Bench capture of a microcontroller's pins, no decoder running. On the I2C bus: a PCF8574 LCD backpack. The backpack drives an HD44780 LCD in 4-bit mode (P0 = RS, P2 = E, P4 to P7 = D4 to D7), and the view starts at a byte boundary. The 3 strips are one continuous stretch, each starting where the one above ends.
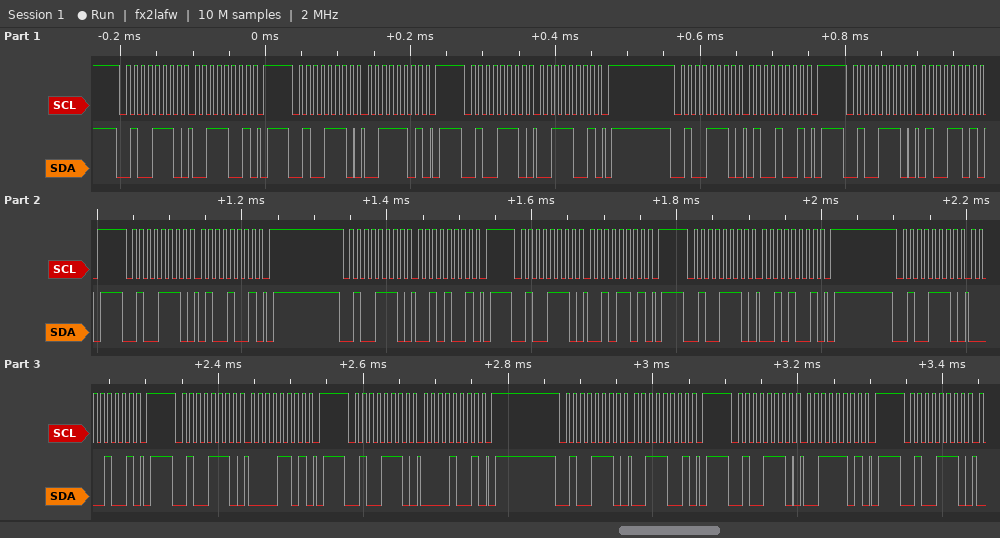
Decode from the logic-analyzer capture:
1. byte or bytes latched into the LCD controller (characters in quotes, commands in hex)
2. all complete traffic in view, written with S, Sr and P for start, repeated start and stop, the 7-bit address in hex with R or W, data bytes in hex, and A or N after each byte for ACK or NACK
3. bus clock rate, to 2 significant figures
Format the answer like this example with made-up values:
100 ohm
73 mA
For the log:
'4' ' '
S 27W A 39 A P S 27W A 3D A P S 27W A 39 A P S 27W A 49 A P S 27W A 4D A P S 27W A 49 A P S 27W A 29 A P S 27W A 2D A P S 27W A 29 A P S 27W A 09 A P S 27W A 0D A P S 27W A 09 A P S 27W A 39 A P S 27W A 3D A P S 27W A
100 kHz
